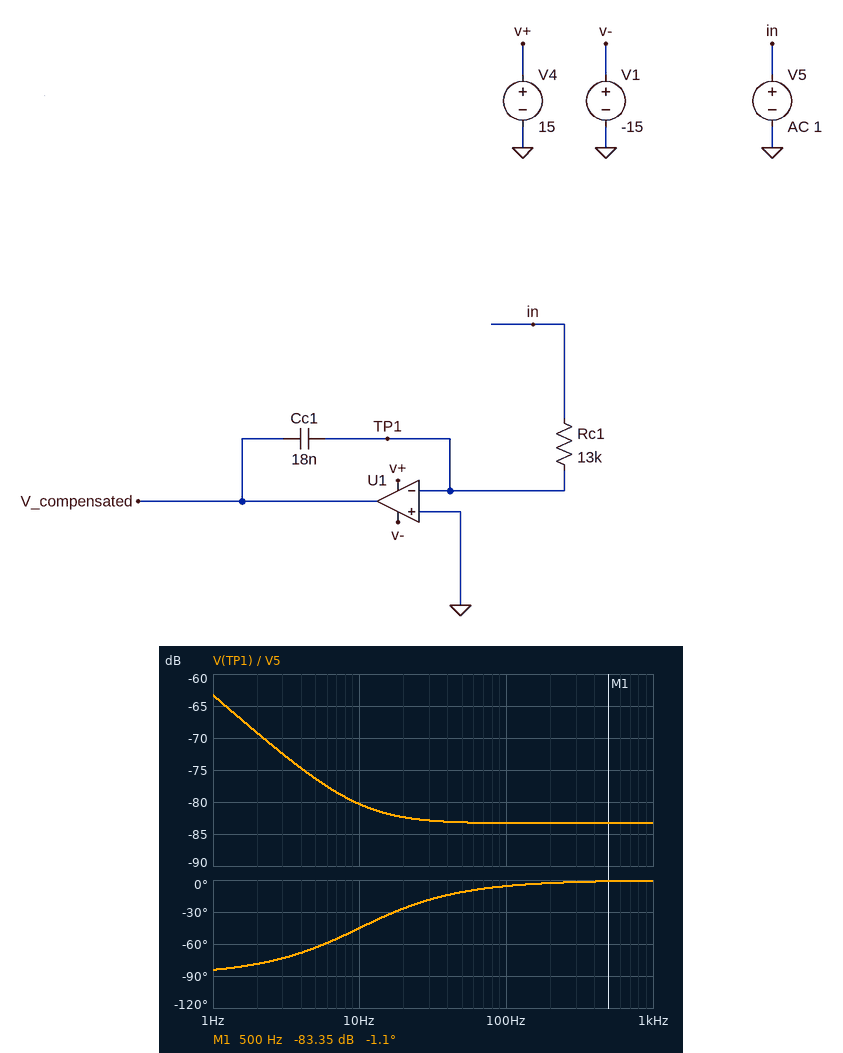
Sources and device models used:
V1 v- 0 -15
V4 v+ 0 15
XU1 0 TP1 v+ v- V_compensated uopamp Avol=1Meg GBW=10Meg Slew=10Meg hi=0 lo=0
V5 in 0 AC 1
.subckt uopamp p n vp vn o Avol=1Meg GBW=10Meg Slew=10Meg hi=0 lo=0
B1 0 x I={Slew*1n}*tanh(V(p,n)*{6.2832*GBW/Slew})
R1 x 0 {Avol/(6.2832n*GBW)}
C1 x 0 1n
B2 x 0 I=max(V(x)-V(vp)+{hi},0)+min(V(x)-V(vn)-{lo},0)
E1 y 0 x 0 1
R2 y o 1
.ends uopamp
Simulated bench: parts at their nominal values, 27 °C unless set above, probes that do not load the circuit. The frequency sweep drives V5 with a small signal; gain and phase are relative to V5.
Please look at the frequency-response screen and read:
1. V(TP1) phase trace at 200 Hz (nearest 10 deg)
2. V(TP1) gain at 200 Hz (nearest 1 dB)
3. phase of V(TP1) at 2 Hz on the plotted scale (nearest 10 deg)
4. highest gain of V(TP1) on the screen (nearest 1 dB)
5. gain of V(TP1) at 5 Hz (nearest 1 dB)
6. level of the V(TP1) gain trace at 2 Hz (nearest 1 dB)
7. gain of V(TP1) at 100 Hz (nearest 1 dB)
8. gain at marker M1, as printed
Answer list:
0 deg
-83 dB
-80 deg
-63 dB
-76 dB
-69 dB
-83 dB
-83.35 dB
